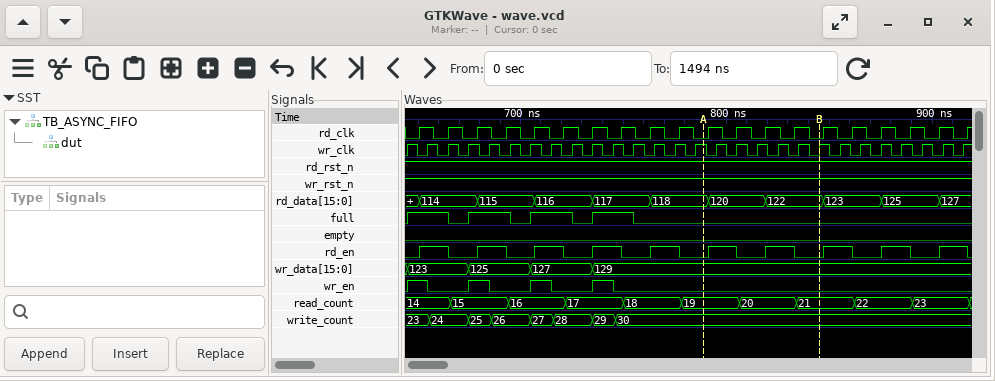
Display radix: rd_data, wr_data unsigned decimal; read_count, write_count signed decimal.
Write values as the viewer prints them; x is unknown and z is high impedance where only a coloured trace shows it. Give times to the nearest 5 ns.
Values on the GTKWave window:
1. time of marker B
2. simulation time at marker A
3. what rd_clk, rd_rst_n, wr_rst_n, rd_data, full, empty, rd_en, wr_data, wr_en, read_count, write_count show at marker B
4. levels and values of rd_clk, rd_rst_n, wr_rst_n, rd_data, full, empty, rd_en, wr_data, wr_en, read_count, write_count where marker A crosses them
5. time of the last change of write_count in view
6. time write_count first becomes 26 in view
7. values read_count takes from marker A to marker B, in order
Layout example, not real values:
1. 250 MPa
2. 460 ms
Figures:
1. 845 ns
2. 790 ns
3. rd_clk=0, rd_rst_n=1, wr_rst_n=1, rd_data=122, full=0, empty=0, rd_en=0, wr_data=129, wr_en=0, read_count=21, write_count=30
4. rd_clk=0, rd_rst_n=1, wr_rst_n=1, rd_data=118, full=0, empty=0, rd_en=0, wr_data=129, wr_en=0, read_count=19, write_count=30
5. 745 ns
6. 685 ns
7. 19, 20, 21
